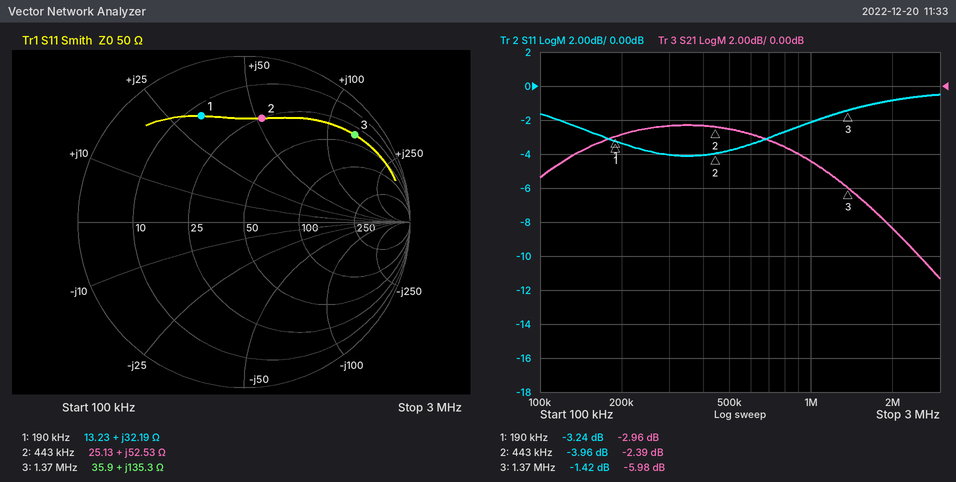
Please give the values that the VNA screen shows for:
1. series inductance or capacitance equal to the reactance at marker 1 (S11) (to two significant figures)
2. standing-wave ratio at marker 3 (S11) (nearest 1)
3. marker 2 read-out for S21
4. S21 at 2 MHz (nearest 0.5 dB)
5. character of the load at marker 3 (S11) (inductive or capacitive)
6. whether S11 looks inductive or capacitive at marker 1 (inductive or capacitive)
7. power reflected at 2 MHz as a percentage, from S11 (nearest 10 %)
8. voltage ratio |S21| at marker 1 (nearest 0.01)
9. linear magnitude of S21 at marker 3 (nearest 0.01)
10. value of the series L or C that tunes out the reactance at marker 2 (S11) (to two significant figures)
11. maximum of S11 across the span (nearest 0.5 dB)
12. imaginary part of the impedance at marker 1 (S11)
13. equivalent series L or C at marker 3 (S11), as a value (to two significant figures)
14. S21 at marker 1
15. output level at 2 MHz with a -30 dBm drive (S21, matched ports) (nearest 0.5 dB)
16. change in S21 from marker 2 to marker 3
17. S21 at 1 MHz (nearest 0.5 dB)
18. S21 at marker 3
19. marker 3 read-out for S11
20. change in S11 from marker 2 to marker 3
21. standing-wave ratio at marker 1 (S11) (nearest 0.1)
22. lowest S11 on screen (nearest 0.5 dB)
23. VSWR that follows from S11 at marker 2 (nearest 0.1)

27 µH
12
-2.39 dB
-8.5 dB
inductive
inductive
80 %
0.71
0.50
6.8 nF
-0.5 dB
+32.19 Ω
16 µH
-2.96 dB
-38.5 dBm
-3.59 dB
-4.5 dB
-5.98 dB
-1.42 dB
2.54 dB
5.4
-4.0 dB
4.5
